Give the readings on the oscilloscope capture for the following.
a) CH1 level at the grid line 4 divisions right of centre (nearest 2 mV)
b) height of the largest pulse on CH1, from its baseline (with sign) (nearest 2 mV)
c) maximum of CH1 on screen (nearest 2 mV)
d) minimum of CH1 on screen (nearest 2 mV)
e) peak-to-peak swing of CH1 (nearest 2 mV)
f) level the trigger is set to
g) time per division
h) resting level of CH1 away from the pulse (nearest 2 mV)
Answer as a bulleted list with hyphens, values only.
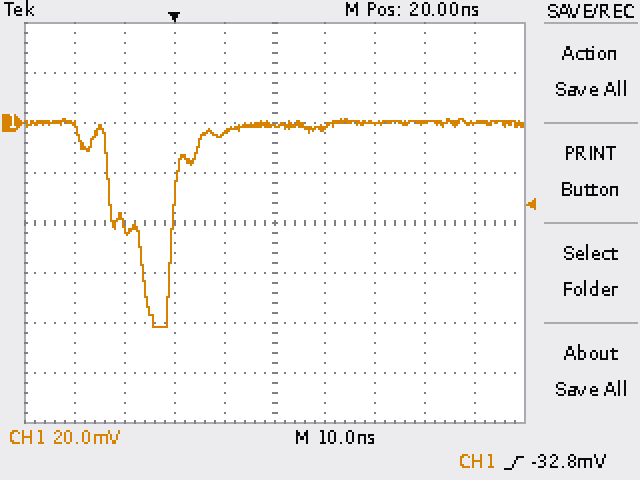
- 0 mV
- -82 mV
- 2 mV
- -82 mV
- 84 mV
- -32.8 mV
- 10 ns
- 0 mV
